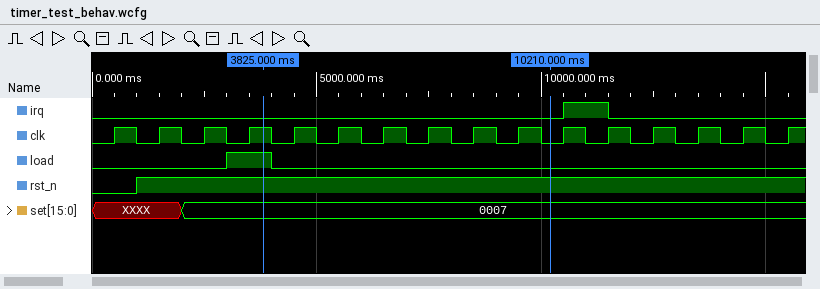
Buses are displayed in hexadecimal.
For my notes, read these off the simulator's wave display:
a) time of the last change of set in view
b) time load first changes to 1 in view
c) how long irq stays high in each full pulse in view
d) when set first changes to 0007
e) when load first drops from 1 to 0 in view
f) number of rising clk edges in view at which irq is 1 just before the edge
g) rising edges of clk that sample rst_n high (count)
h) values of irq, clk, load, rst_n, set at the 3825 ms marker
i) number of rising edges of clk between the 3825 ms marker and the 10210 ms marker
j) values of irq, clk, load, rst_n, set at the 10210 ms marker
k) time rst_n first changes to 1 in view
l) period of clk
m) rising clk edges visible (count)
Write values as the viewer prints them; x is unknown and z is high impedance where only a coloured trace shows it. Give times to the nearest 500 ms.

2000 ms
3000 ms
1000 ms
2000 ms
4000 ms
1
15
irq=0, clk=1, load=1, rst_n=1, set=0007
6
irq=0, clk=0, load=0, rst_n=1, set=0007
1000 ms
1000 ms
16
